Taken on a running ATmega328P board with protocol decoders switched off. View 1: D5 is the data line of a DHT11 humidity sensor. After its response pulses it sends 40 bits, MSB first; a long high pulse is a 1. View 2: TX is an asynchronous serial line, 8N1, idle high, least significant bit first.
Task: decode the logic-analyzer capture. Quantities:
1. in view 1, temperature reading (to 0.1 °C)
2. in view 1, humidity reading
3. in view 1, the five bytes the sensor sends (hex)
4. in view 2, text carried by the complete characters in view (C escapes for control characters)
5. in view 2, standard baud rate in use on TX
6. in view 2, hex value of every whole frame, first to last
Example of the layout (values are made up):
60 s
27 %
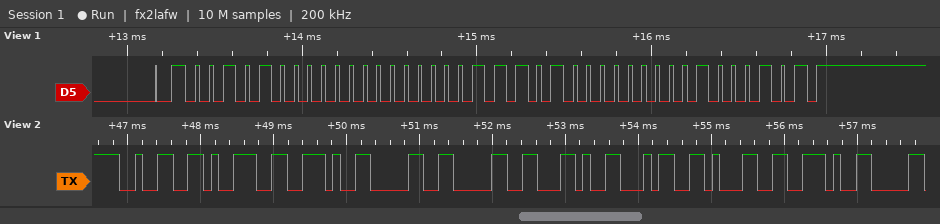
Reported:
29.0 °C
40 %
28 00 1D 00 45
"29.00,41."
9600 baud
32 39 2E 30 30 2C 34 31 2E
